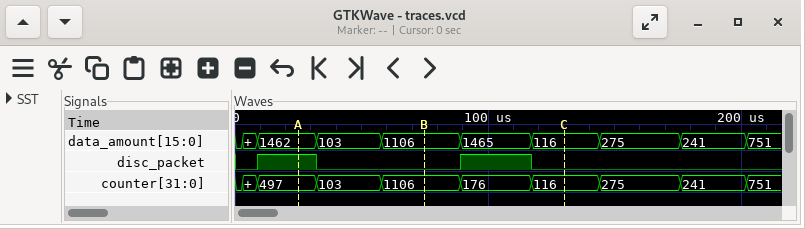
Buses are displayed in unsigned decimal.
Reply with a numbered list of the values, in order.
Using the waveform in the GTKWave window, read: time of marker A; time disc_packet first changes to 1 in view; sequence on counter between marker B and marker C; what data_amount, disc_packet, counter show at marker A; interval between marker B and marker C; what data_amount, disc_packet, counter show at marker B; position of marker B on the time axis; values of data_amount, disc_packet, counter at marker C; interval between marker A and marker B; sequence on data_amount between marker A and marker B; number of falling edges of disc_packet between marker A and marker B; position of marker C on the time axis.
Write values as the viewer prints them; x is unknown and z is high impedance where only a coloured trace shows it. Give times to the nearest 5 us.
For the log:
1. 25 us
2. 10 us
3. 1106, 176, 116
4. data_amount=1462, disc_packet=1, counter=497
5. 55 us
6. data_amount=1106, disc_packet=0, counter=1106
7. 75 us
8. data_amount=116, disc_packet=0, counter=116
9. 50 us
10. 1462, 103, 1106
11. 1
12. 130 us
